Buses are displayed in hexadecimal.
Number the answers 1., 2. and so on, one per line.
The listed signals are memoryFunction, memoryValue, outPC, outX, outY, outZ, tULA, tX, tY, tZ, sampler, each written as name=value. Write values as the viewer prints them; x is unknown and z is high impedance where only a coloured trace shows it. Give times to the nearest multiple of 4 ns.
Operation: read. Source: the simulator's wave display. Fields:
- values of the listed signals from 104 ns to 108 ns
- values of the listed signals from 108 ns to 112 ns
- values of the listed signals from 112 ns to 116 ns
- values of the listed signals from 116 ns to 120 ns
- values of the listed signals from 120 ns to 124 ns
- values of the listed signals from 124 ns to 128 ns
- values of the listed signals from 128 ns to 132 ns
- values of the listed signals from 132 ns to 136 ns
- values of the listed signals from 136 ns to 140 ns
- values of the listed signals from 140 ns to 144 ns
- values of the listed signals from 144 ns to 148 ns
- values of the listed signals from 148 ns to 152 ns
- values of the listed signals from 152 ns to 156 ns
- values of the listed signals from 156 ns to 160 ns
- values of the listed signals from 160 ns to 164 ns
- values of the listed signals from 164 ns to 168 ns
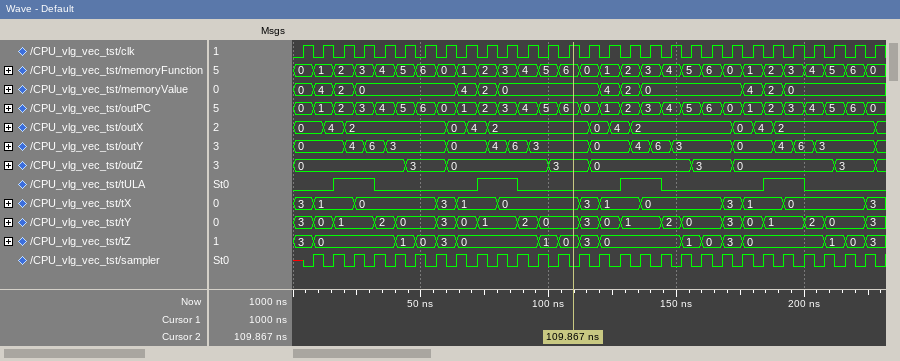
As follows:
1. memoryFunction=6, memoryValue=0, outPC=6, outX=2, outY=3, outZ=3, tULA=0, tX=0, tY=0, tZ=0, sampler=1
2. memoryFunction=6, memoryValue=0, outPC=6, outX=2, outY=3, outZ=3, tULA=0, tX=0, tY=0, tZ=0, sampler=0
3. memoryFunction=0, memoryValue=0, outPC=0, outX=2, outY=3, outZ=3, tULA=0, tX=3, tY=3, tZ=3, sampler=1
4. memoryFunction=0, memoryValue=0, outPC=0, outX=0, outY=0, outZ=0, tULA=0, tX=3, tY=3, tZ=3, sampler=0
5. memoryFunction=1, memoryValue=4, outPC=1, outX=0, outY=0, outZ=0, tULA=0, tX=1, tY=0, tZ=0, sampler=1
6. memoryFunction=1, memoryValue=4, outPC=1, outX=4, outY=0, outZ=0, tULA=0, tX=1, tY=0, tZ=0, sampler=0
7. memoryFunction=2, memoryValue=2, outPC=2, outX=4, outY=0, outZ=0, tULA=1, tX=1, tY=1, tZ=0, sampler=1
8. memoryFunction=2, memoryValue=2, outPC=2, outX=2, outY=4, outZ=0, tULA=1, tX=1, tY=1, tZ=0, sampler=0
9. memoryFunction=3, memoryValue=0, outPC=3, outX=2, outY=4, outZ=0, tULA=1, tX=0, tY=1, tZ=0, sampler=1
10. memoryFunction=3, memoryValue=0, outPC=3, outX=2, outY=6, outZ=0, tULA=1, tX=0, tY=1, tZ=0, sampler=0
11. memoryFunction=4, memoryValue=0, outPC=4, outX=2, outY=6, outZ=0, tULA=0, tX=0, tY=2, tZ=0, sampler=1
12. memoryFunction=4, memoryValue=0, outPC=4, outX=2, outY=3, outZ=0, tULA=0, tX=0, tY=2, tZ=0, sampler=0
13. memoryFunction=5, memoryValue=0, outPC=5, outX=2, outY=3, outZ=0, tULA=0, tX=0, tY=0, tZ=1, sampler=1
14. memoryFunction=5, memoryValue=0, outPC=5, outX=2, outY=3, outZ=3, tULA=0, tX=0, tY=0, tZ=1, sampler=0
15. memoryFunction=6, memoryValue=0, outPC=6, outX=2, outY=3, outZ=3, tULA=0, tX=0, tY=0, tZ=0, sampler=1
16. memoryFunction=6, memoryValue=0, outPC=6, outX=2, outY=3, outZ=3, tULA=0, tX=0, tY=0, tZ=0, sampler=0
